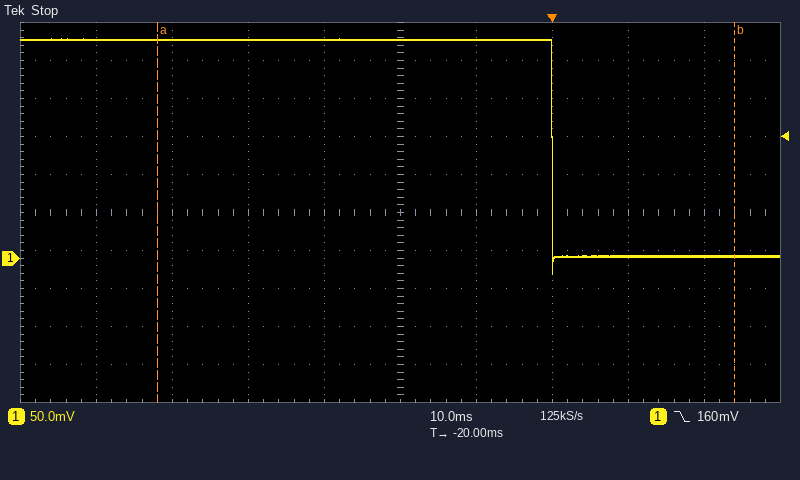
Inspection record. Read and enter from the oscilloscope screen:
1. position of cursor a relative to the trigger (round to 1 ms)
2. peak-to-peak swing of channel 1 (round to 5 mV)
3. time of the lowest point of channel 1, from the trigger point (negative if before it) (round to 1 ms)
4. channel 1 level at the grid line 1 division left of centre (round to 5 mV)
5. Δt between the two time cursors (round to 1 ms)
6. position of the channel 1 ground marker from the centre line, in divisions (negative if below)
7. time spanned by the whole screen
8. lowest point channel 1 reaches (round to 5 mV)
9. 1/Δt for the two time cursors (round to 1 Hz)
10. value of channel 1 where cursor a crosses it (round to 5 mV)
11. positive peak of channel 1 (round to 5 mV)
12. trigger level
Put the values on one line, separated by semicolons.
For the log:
-52 ms; 310 mV; 0 ms; 290 mV; 76 ms; -1.2 div; 100 ms; -20 mV; 13 Hz; 290 mV; 290 mV; 160 mV
